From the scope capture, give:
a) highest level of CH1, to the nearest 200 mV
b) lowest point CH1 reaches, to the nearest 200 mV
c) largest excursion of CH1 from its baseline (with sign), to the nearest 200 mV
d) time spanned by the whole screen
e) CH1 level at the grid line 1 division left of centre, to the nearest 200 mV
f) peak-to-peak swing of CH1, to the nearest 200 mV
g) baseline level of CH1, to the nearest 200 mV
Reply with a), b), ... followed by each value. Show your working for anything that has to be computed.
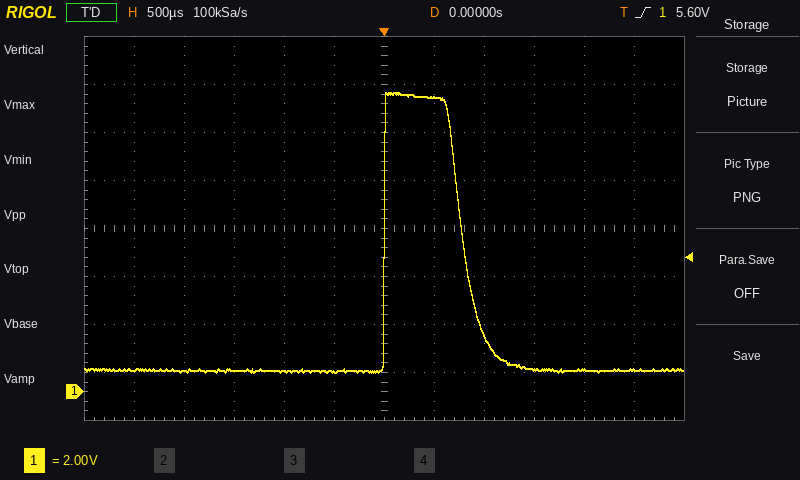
a) 12.4 V
b) 800 mV
c) 12.4 V − (800 mV) = +11.6 V
d) 6 ms
e) 800 mV
f) 12.4 V − (800 mV) = 11.6 V
g) 800 mV
